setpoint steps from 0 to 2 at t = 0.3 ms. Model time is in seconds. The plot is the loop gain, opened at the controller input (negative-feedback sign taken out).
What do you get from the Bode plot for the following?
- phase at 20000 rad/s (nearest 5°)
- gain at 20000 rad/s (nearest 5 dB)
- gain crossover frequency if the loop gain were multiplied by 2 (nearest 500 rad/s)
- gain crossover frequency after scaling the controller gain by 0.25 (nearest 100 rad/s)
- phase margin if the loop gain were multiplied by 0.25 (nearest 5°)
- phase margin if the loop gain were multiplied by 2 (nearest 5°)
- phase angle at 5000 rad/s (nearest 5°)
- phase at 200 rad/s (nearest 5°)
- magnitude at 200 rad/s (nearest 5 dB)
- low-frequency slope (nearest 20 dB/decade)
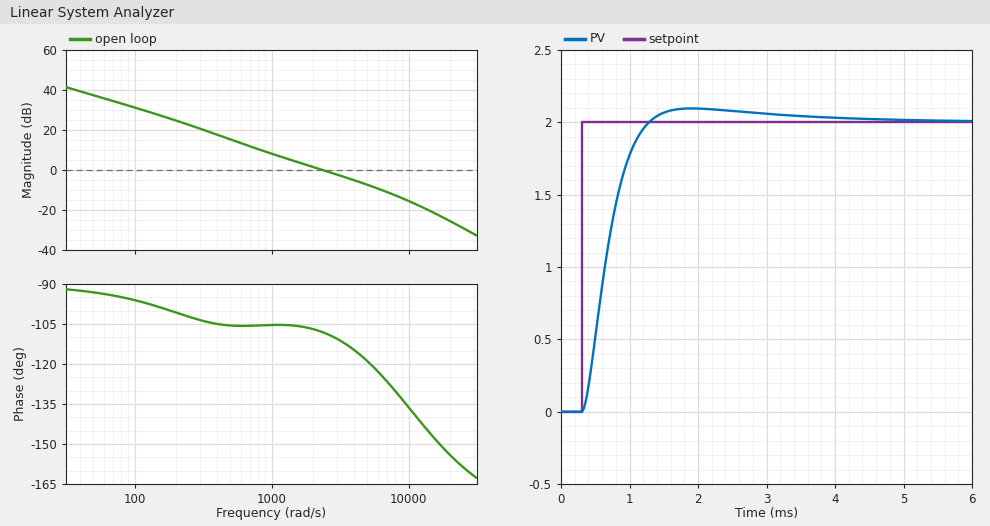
-155°
-25 dB
4500 rad/s
700 rad/s
75°
65°
-120°
-100°
25 dB
-20 dB/decade
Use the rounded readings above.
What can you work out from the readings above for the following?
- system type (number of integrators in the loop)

1
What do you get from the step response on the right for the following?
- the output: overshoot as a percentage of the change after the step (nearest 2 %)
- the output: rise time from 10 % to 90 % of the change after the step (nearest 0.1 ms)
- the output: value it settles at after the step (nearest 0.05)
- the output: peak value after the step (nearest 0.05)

4 %
0.6 ms
2.00
2.10
